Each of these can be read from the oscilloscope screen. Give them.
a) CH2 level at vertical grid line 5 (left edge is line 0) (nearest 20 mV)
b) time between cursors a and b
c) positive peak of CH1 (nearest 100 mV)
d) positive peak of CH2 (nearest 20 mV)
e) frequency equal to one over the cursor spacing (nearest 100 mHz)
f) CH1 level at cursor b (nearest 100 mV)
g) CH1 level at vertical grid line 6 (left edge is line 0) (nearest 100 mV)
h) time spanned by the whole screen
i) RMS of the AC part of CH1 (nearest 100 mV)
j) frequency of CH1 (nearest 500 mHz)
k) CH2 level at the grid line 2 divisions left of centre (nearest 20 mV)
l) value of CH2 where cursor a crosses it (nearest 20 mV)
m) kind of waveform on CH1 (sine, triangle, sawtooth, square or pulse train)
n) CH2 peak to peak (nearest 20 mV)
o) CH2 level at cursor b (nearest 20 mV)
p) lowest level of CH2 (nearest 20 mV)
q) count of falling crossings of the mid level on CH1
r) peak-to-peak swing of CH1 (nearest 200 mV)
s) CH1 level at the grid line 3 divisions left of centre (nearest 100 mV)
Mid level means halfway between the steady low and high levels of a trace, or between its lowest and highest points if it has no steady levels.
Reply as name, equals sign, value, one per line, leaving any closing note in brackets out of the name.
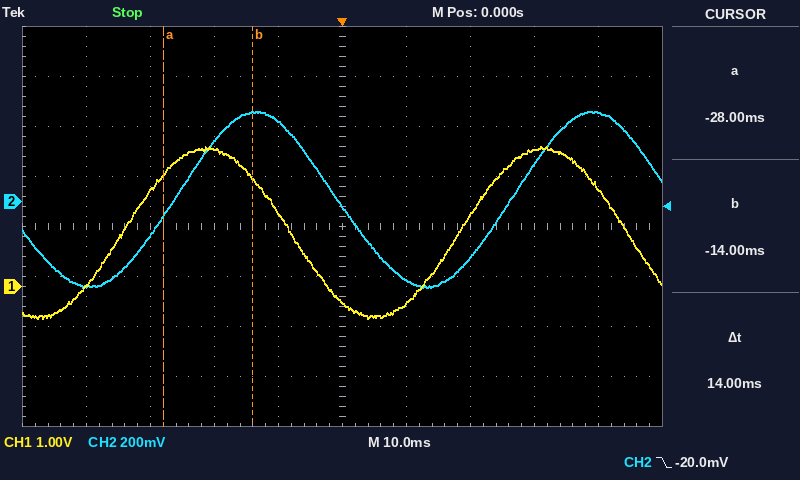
CH2 level at vertical grid line 5 (left edge is line 0) = -20 mV
time between cursors a and b = 14 ms
positive peak of CH1 = 2.8 V
positive peak of CH2 = 360 mV
frequency equal to one over the cursor spacing = 71.4 Hz
CH1 level at cursor b = 2.2 V
CH1 level at vertical grid line 6 (left edge is line 0) = -300 mV
time spanned by the whole screen = 100 ms
RMS of the AC part of CH1 = 1.2 V
frequency of CH1 = 19.0 Hz
CH2 level at the grid line 2 divisions left of centre = 240 mV
value of CH2 where cursor a crosses it = -60 mV
kind of waveform on CH1 = sine
CH2 peak to peak = 700 mV
CH2 level at cursor b = 360 mV
lowest level of CH2 = -340 mV
count of falling crossings of the mid level on CH1 = 2
peak-to-peak swing of CH1 = 3.4 V
CH1 level at the grid line 3 divisions left of centre = 1.9 V
